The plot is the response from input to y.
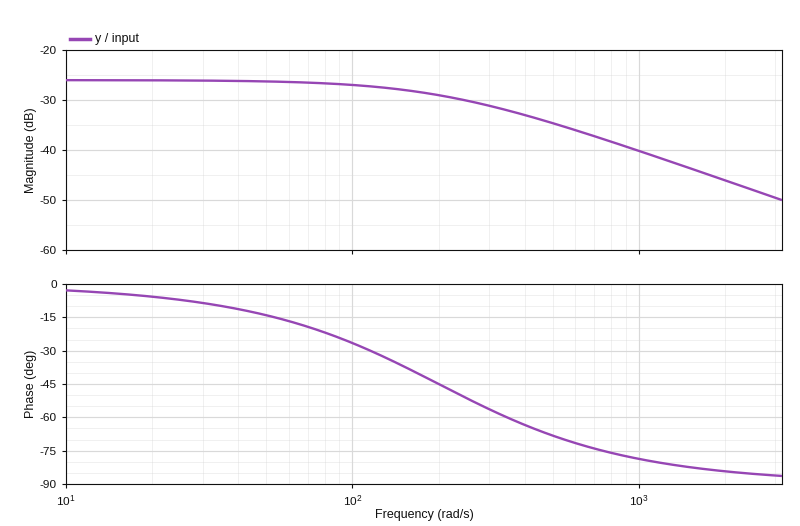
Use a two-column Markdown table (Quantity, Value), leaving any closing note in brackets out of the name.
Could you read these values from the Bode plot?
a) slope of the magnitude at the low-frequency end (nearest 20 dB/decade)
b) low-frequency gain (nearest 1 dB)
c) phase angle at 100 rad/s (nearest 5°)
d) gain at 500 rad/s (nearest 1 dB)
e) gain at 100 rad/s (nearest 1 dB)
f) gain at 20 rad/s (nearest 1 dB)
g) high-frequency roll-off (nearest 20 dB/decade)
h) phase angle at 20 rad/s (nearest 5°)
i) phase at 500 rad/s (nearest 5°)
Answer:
| Quantity | Value |
|---|---|
| slope of the magnitude at the low-frequency end | 0 dB/decade |
| low-frequency gain | -26 dB |
| phase angle at 100 rad/s | -25° |
| gain at 500 rad/s | -35 dB |
| gain at 100 rad/s | -27 dB |
| gain at 20 rad/s | -26 dB |
| high-frequency roll-off | -20 dB/decade |
| phase angle at 20 rad/s | -5° |
| phase at 500 rad/s | -70° |
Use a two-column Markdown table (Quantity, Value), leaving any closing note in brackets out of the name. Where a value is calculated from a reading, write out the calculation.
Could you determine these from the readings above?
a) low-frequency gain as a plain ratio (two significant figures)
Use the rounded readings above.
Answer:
| Quantity | Value |
|---|---|
| low-frequency gain as a plain ratio | 10^(-26 / 20) = 0.050 |
